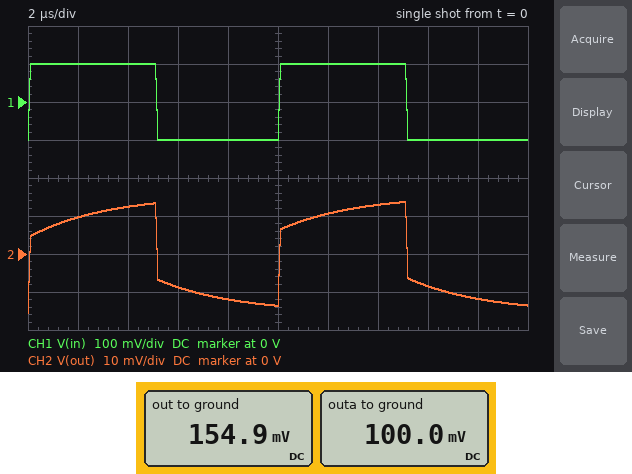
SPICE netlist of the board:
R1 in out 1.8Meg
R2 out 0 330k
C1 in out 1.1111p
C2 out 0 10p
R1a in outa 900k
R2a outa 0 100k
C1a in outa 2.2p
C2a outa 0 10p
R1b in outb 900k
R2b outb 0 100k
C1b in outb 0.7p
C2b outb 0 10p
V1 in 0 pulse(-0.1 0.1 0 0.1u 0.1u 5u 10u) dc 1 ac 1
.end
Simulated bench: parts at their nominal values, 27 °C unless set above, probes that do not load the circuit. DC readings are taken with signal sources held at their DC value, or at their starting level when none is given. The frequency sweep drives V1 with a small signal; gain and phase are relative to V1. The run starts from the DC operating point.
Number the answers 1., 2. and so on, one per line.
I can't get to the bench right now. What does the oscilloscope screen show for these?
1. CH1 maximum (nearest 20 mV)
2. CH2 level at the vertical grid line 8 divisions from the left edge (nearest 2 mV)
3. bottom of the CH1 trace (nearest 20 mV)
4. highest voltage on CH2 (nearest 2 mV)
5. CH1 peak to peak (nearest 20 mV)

1. 100 mV
2. -8 mV
3. -100 mV
4. 14 mV
5. 200 mV
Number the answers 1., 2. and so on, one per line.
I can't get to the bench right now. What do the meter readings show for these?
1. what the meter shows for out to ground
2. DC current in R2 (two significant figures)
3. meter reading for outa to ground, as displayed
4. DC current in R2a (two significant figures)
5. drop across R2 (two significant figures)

1. 154.9 mV
2. 470 nA
3. 100.0 mV
4. 1.0 µA
5. 150 mV
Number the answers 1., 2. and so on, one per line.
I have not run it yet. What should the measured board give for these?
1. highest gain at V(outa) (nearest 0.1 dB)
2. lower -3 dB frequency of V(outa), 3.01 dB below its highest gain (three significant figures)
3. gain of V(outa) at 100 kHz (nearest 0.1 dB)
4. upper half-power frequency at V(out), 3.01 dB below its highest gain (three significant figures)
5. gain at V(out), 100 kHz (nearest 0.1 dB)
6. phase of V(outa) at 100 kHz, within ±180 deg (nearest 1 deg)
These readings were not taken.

1. -14.9 dB
2. 89.9 kHz
3. -17.6 dB
4. 126 kHz
5. -18.9 dB
6. 17 deg
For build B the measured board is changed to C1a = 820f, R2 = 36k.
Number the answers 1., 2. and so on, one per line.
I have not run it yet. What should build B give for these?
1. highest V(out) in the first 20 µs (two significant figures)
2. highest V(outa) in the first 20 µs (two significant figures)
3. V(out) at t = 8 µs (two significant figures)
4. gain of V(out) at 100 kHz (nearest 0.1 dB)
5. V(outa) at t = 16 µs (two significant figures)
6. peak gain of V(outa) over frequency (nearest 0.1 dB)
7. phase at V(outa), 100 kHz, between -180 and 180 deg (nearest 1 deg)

1. 16 mV
2. 10 mV
3. -2.0 mV
4. -30.3 dB
5. -8.0 mV
6. -20.0 dB
7. -7 deg
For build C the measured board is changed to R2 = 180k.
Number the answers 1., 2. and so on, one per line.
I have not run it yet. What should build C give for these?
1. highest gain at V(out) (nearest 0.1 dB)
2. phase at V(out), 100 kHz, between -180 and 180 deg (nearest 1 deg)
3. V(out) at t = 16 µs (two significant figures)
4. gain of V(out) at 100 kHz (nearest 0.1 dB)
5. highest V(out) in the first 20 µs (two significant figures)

1. -20.0 dB
2. 3 deg
3. -10 mV
4. -20.3 dB
5. 11 mV
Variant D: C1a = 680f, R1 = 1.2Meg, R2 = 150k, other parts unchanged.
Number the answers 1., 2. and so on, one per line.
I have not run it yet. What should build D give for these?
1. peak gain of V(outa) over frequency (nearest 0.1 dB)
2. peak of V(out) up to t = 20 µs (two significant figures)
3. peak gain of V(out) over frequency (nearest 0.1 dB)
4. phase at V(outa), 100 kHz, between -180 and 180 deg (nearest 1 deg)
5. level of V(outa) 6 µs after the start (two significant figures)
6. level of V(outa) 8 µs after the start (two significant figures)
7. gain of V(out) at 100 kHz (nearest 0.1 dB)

1. -20.0 dB
2. 11 mV
3. -19.1 dB
4. -10 deg
5. -7.0 mV
6. -9.6 mV
7. -19.5 dB
